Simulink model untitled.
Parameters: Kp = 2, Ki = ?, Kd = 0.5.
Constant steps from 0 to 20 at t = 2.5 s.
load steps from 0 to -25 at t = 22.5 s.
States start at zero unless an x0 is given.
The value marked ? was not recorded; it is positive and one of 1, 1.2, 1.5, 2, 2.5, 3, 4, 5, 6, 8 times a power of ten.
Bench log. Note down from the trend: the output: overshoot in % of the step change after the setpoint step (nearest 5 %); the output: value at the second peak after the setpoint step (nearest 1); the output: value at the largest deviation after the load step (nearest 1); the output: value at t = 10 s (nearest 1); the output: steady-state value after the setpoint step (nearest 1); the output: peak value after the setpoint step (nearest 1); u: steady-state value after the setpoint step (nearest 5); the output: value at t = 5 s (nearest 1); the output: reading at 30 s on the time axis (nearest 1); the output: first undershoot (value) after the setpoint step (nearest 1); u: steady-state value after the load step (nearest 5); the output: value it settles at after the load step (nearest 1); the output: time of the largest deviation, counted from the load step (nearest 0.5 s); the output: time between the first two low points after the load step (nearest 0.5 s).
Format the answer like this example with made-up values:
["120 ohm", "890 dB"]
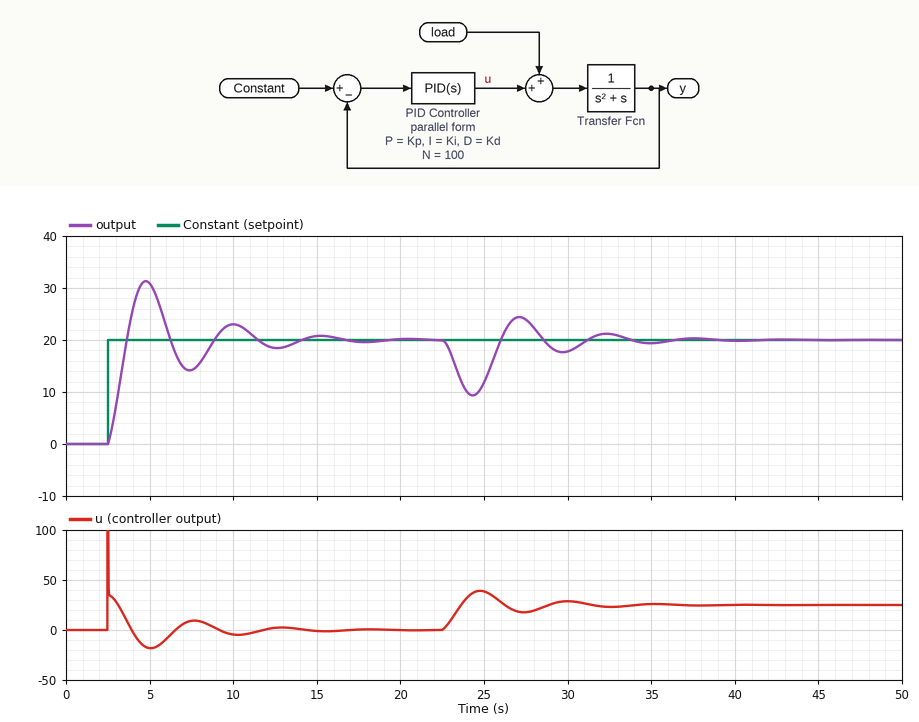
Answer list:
["55 %", "23", "9", "23", "20", "31", "0", "31", "18", "14", "25", "20", "2.0 s", "5.5 s"]
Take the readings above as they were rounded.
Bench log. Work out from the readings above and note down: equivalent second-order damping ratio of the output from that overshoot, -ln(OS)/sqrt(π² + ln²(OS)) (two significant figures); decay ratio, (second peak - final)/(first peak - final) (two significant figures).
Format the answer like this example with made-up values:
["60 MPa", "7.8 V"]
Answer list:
["0.19", "0.27"]
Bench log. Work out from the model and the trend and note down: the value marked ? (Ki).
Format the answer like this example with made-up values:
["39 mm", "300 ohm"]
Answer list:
["1.5"]
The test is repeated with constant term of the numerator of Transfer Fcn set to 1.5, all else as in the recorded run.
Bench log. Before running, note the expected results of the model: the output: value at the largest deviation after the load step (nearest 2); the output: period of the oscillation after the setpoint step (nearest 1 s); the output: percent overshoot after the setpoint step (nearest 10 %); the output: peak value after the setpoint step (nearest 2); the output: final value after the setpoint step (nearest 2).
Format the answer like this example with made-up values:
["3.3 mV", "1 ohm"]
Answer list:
["8", "4 s", "50 %", "30", "20"]
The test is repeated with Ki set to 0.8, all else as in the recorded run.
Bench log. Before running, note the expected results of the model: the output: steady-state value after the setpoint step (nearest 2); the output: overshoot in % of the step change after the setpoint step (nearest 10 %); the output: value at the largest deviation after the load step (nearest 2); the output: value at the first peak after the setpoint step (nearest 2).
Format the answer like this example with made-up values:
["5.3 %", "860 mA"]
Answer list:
["20", "40 %", "8", "28"]
